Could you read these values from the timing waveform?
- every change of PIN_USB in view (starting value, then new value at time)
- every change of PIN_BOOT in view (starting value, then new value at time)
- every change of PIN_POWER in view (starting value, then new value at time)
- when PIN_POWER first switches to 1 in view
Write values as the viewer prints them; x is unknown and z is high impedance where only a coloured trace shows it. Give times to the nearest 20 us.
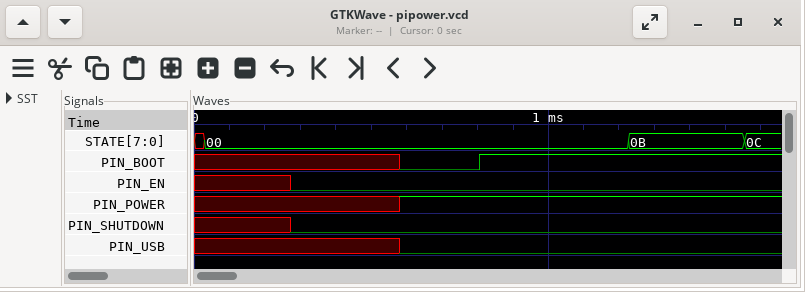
x, 0 at 580 us
x, 0 at 580 us, 1 at 800 us
x, 1 at 580 us
580 us
